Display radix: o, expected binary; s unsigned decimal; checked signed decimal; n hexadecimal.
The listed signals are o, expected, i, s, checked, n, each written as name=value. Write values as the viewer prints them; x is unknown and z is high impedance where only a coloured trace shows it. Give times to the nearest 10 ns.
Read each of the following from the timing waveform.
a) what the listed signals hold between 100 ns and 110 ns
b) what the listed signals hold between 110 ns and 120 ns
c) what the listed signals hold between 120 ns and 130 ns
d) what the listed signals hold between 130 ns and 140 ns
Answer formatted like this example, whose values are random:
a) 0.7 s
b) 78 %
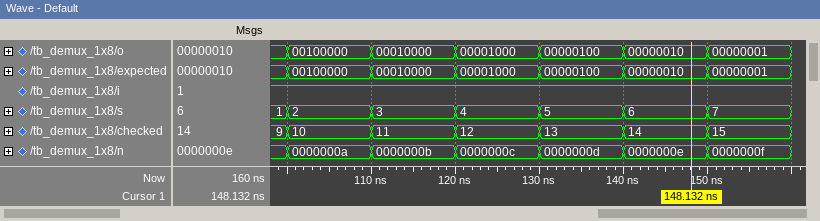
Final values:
a) o=00100000, expected=00100000, i=1, s=2, checked=10, n=0000000a
b) o=00010000, expected=00010000, i=1, s=3, checked=11, n=0000000b
c) o=00001000, expected=00001000, i=1, s=4, checked=12, n=0000000c
d) o=00000100, expected=00000100, i=1, s=5, checked=13, n=0000000d
